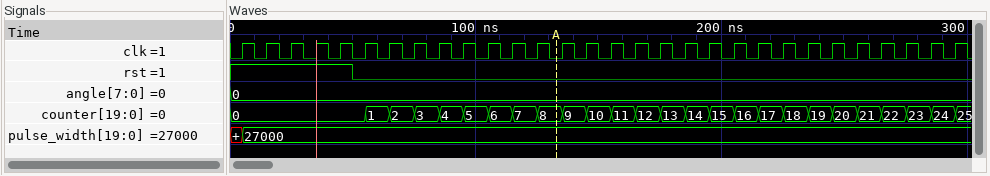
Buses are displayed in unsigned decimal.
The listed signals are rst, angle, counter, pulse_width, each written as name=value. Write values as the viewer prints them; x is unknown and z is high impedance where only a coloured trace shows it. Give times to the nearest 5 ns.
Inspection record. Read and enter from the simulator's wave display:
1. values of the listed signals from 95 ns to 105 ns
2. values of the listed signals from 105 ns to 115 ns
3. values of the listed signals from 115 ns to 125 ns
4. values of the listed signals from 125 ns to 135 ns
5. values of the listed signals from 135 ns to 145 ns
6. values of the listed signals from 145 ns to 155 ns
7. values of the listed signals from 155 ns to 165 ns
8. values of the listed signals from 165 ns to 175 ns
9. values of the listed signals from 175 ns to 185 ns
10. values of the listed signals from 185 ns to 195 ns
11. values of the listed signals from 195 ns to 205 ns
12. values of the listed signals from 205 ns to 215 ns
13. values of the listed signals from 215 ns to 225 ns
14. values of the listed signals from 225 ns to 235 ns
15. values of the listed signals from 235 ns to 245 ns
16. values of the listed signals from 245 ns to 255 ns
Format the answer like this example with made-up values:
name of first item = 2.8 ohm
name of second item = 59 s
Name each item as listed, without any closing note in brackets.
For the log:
values of the listed signals from 95 ns to 105 ns = rst=0, angle=0, counter=5, pulse_width=27000
values of the listed signals from 105 ns to 115 ns = rst=0, angle=0, counter=6, pulse_width=27000
values of the listed signals from 115 ns to 125 ns = rst=0, angle=0, counter=7, pulse_width=27000
values of the listed signals from 125 ns to 135 ns = rst=0, angle=0, counter=8, pulse_width=27000
values of the listed signals from 135 ns to 145 ns = rst=0, angle=0, counter=9, pulse_width=27000
values of the listed signals from 145 ns to 155 ns = rst=0, angle=0, counter=10, pulse_width=27000
values of the listed signals from 155 ns to 165 ns = rst=0, angle=0, counter=11, pulse_width=27000
values of the listed signals from 165 ns to 175 ns = rst=0, angle=0, counter=12, pulse_width=27000
values of the listed signals from 175 ns to 185 ns = rst=0, angle=0, counter=13, pulse_width=27000
values of the listed signals from 185 ns to 195 ns = rst=0, angle=0, counter=14, pulse_width=27000
values of the listed signals from 195 ns to 205 ns = rst=0, angle=0, counter=15, pulse_width=27000
values of the listed signals from 205 ns to 215 ns = rst=0, angle=0, counter=16, pulse_width=27000
values of the listed signals from 215 ns to 225 ns = rst=0, angle=0, counter=17, pulse_width=27000
values of the listed signals from 225 ns to 235 ns = rst=0, angle=0, counter=18, pulse_width=27000
values of the listed signals from 235 ns to 245 ns = rst=0, angle=0, counter=19, pulse_width=27000
values of the listed signals from 245 ns to 255 ns = rst=0, angle=0, counter=20, pulse_width=27000
